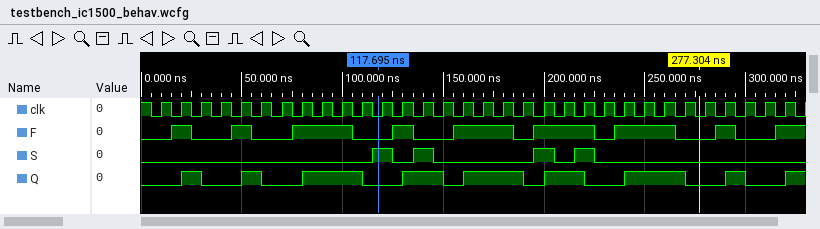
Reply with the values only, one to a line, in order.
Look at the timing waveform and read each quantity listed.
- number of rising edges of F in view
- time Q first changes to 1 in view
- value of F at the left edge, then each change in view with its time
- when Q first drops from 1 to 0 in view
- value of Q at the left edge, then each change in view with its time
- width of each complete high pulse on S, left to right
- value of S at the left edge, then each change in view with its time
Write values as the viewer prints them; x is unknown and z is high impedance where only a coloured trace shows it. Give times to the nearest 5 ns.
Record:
9
20 ns
0, 1 at 15 ns, 0 at 25 ns, 1 at 45 ns, 0 at 55 ns, 1 at 75 ns, 0 at 105 ns, 1 at 125 ns, 0 at 135 ns, 1 at 155 ns, 0 at 185 ns, 1 at 195 ns, 0 at 225 ns, 1 at 235 ns, 0 at 265 ns, 1 at 285 ns, 0 at 295 ns, 1 at 315 ns
30 ns
0, 1 at 20 ns, 0 at 30 ns, 1 at 50 ns, 0 at 60 ns, 1 at 80 ns, 0 at 110 ns, 1 at 130 ns, 0 at 150 ns, 1 at 160 ns, 0 at 190 ns, 1 at 200 ns, 0 at 220 ns, 1 at 240 ns, 0 at 270 ns, 1 at 290 ns, 0 at 300 ns, 1 at 320 ns
10 ns, 10 ns, 10 ns, 10 ns
0, 1 at 115 ns, 0 at 125 ns, 1 at 135 ns, 0 at 145 ns, 1 at 195 ns, 0 at 205 ns, 1 at 215 ns, 0 at 225 ns
